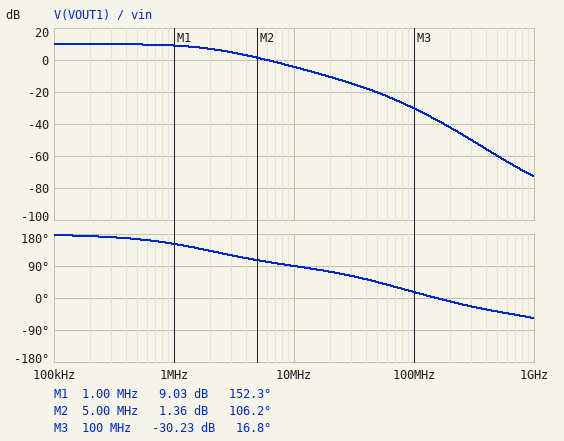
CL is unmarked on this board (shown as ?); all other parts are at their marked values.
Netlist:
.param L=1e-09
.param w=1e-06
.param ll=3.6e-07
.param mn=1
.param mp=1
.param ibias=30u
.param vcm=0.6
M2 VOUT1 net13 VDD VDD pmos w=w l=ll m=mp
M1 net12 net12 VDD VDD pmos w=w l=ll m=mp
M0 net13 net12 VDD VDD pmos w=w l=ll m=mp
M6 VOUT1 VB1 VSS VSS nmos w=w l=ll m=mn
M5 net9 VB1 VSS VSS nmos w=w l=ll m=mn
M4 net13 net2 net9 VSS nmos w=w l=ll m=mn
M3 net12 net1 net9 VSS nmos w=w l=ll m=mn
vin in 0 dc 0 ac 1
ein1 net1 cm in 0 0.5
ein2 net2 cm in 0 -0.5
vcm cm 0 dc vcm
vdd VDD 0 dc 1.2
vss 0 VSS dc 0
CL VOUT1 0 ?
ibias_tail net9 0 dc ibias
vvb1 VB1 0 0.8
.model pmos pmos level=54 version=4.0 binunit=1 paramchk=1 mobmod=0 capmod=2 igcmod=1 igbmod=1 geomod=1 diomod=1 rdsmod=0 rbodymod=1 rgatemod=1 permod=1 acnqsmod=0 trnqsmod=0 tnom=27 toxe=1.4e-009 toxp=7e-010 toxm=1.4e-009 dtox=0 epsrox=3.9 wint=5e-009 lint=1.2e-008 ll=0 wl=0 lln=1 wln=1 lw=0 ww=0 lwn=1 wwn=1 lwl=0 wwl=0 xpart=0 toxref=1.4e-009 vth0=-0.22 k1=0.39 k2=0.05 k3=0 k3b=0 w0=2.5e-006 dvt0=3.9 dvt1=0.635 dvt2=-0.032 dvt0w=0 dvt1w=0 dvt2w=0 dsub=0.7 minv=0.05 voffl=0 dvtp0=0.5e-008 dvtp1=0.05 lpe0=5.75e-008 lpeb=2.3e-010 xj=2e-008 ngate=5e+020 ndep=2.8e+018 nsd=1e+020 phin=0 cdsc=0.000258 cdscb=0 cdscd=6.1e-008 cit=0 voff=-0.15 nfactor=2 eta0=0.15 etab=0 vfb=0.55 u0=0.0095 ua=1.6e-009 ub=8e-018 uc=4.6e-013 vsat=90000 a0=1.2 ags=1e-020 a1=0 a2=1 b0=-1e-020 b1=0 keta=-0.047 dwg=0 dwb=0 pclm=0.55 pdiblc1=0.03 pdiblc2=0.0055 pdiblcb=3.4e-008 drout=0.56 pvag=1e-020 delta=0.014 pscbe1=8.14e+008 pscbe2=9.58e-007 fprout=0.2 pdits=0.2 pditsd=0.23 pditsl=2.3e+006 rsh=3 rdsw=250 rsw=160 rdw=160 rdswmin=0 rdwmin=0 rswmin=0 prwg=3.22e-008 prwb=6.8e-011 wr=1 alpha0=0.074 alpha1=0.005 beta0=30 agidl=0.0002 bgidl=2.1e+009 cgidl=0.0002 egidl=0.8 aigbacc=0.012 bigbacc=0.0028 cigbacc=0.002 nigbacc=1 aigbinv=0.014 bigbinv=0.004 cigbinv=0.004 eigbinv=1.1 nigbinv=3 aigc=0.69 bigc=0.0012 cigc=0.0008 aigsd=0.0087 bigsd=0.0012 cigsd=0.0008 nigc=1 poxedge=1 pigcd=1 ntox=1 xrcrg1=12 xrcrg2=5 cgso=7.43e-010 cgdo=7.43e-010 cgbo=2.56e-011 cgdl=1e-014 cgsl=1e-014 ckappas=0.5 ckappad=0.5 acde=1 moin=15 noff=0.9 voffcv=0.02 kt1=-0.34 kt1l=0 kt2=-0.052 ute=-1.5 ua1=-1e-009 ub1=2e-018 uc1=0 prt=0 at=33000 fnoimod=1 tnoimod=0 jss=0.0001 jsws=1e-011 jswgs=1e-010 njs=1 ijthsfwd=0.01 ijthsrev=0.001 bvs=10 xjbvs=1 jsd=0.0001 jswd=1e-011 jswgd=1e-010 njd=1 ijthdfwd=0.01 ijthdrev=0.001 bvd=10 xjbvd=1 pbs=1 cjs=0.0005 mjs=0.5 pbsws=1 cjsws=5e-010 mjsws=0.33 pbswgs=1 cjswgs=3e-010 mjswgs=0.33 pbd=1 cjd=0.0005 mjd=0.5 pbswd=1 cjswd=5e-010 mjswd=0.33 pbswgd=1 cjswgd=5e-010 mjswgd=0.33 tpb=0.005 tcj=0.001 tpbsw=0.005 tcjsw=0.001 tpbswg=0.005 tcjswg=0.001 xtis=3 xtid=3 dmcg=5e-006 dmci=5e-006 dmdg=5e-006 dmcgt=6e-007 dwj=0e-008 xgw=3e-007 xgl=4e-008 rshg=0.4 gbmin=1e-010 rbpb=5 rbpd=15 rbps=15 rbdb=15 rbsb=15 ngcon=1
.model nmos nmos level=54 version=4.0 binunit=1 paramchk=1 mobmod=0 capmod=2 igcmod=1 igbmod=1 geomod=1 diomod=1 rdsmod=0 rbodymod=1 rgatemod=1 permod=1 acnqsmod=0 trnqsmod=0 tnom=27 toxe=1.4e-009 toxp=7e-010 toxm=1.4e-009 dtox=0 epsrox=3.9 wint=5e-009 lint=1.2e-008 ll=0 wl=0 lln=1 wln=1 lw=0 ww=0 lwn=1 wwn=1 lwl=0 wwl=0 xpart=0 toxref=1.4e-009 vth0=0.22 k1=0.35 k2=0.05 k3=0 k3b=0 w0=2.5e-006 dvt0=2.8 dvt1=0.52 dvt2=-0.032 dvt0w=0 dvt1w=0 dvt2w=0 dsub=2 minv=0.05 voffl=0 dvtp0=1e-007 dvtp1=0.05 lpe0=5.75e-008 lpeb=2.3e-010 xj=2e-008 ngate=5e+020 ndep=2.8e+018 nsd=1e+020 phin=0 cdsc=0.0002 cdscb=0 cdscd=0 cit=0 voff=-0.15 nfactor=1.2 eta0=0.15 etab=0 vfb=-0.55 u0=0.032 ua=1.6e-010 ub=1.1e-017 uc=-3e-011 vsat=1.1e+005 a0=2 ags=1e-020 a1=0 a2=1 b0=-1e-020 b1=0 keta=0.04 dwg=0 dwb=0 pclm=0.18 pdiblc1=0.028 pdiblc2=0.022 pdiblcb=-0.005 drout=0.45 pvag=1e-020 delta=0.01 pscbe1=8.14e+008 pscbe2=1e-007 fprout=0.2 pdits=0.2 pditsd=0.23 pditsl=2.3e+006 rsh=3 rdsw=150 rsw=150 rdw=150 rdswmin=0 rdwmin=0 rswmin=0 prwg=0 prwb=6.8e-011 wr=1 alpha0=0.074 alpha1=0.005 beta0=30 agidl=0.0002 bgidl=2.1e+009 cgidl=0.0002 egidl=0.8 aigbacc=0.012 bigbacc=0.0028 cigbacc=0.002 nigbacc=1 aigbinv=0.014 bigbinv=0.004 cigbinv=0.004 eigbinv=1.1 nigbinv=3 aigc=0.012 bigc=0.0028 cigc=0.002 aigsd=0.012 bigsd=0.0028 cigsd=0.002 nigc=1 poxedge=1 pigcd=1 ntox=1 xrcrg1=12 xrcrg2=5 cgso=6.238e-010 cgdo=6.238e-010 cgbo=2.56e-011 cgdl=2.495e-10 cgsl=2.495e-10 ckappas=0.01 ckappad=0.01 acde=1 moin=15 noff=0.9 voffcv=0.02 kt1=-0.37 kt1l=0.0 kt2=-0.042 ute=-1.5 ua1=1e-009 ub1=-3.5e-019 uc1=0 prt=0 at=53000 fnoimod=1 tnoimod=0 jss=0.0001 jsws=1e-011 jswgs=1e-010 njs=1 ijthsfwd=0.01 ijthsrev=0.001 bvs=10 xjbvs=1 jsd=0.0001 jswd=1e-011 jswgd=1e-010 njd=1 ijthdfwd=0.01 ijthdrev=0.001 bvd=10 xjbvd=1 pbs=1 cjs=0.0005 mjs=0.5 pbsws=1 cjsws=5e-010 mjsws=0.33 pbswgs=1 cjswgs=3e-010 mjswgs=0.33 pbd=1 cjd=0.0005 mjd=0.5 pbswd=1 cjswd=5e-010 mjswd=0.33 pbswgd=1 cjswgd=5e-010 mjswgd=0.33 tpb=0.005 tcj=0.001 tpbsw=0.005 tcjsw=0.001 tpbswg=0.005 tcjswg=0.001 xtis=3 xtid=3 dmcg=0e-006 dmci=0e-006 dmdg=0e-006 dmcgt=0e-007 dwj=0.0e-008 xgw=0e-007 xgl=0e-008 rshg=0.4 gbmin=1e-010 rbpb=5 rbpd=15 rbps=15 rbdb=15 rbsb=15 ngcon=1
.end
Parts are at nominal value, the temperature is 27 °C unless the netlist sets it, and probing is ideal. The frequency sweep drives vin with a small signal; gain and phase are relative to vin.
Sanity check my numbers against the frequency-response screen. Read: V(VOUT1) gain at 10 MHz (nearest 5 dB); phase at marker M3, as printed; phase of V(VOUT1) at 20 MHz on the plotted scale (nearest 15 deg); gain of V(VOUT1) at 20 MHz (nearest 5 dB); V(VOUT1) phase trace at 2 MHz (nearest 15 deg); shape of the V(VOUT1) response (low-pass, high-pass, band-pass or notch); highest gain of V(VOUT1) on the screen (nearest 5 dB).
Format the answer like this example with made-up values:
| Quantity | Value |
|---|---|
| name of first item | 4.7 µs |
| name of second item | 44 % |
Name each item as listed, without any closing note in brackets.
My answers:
| Quantity | Value |
|---|---|
| V(VOUT1) gain at 10 MHz | -5 dB |
| phase at marker M3, as printed | 16.8 deg |
| phase of V(VOUT1) at 20 MHz on the plotted scale | 75 deg |
| gain of V(VOUT1) at 20 MHz | -10 dB |
| V(VOUT1) phase trace at 2 MHz | 135 deg |
| shape of the V(VOUT1) response | low-pass |
| highest gain of V(VOUT1) on the screen | 10 dB |
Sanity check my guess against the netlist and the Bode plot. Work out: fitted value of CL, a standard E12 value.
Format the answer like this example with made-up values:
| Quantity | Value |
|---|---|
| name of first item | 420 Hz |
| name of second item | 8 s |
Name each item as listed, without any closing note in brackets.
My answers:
| Quantity | Value |
|---|---|
| fitted value of CL, a standard E12 value | 15 pF |
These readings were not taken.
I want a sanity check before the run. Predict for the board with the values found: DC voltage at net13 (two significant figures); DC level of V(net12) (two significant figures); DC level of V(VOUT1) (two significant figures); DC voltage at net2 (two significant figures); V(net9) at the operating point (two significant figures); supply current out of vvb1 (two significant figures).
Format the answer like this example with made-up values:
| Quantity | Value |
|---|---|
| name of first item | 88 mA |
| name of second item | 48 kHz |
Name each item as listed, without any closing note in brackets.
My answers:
| Quantity | Value |
|---|---|
| DC voltage at net13 | 410 mV |
| DC level of V(net12) | 410 mV |
| DC level of V(VOUT1) | 100 mV |
| DC voltage at net2 | 600 mV |
| V(net9) at the operating point | 58 mV |
| supply current out of vvb1 | 3.5 µA |
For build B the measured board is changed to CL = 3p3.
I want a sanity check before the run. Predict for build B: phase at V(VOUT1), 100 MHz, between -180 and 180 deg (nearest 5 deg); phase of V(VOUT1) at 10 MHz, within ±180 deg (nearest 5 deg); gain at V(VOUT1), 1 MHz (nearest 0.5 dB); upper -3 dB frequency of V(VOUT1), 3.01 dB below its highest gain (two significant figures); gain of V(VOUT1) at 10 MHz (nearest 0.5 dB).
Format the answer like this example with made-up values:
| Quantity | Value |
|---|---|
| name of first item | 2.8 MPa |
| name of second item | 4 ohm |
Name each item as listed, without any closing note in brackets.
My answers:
| Quantity | Value |
|---|---|
| phase at V(VOUT1), 100 MHz, between -180 and 180 deg | 20 deg |
| phase of V(VOUT1) at 10 MHz, within ±180 deg | 120 deg |
| gain at V(VOUT1), 1 MHz | 10.0 dB |
| upper -3 dB frequency of V(VOUT1), 3.01 dB below its highest gain | 8.8 MHz |
| gain of V(VOUT1) at 10 MHz | 6.5 dB |
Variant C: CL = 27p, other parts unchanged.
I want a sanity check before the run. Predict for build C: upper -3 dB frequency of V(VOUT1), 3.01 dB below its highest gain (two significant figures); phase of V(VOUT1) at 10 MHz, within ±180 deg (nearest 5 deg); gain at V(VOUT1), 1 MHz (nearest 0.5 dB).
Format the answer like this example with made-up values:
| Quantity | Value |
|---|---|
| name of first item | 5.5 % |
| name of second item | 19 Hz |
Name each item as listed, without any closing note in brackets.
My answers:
| Quantity | Value |
|---|---|
| upper -3 dB frequency of V(VOUT1), 3.01 dB below its highest gain | 1.1 MHz |
| phase of V(VOUT1) at 10 MHz, within ±180 deg | 85 deg |
| gain at V(VOUT1), 1 MHz | 7.5 dB |
